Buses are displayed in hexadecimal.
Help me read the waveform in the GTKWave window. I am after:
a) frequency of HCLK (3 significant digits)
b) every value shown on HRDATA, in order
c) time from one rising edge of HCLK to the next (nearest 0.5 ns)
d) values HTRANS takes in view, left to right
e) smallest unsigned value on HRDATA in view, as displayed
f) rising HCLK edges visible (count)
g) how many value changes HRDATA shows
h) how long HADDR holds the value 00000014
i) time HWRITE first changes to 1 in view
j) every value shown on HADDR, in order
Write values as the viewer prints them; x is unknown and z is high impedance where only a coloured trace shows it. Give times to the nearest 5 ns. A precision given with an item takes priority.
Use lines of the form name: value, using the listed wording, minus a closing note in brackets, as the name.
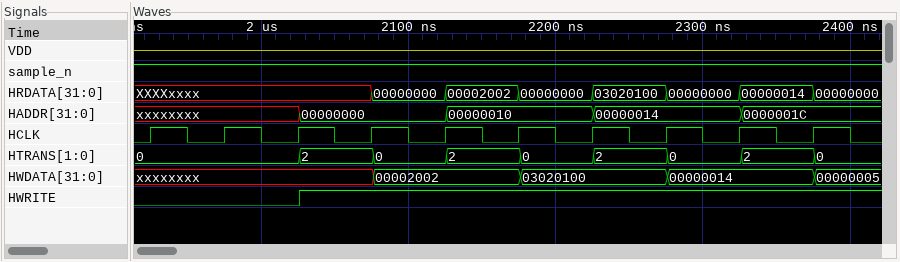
frequency of HCLK: 20.0 MHz
every value shown on HRDATA, in order: XXXXxxxx, 00000000, 00002002, 00000000, 03020100, 00000000, 00000014, 00000000
time from one rising edge of HCLK to the next: 50 ns
values HTRANS takes in view, left to right: 0, 2, 0, 2, 0, 2, 0, 2, 0
smallest unsigned value on HRDATA in view, as displayed: 00000000
rising HCLK edges visible: 10
how many value changes HRDATA shows: 7
how long HADDR holds the value 00000014: 100 ns
time HWRITE first changes to 1 in view: 2025 ns
every value shown on HADDR, in order: xxxxxxxx, 00000000, 00000010, 00000014, 0000001C
